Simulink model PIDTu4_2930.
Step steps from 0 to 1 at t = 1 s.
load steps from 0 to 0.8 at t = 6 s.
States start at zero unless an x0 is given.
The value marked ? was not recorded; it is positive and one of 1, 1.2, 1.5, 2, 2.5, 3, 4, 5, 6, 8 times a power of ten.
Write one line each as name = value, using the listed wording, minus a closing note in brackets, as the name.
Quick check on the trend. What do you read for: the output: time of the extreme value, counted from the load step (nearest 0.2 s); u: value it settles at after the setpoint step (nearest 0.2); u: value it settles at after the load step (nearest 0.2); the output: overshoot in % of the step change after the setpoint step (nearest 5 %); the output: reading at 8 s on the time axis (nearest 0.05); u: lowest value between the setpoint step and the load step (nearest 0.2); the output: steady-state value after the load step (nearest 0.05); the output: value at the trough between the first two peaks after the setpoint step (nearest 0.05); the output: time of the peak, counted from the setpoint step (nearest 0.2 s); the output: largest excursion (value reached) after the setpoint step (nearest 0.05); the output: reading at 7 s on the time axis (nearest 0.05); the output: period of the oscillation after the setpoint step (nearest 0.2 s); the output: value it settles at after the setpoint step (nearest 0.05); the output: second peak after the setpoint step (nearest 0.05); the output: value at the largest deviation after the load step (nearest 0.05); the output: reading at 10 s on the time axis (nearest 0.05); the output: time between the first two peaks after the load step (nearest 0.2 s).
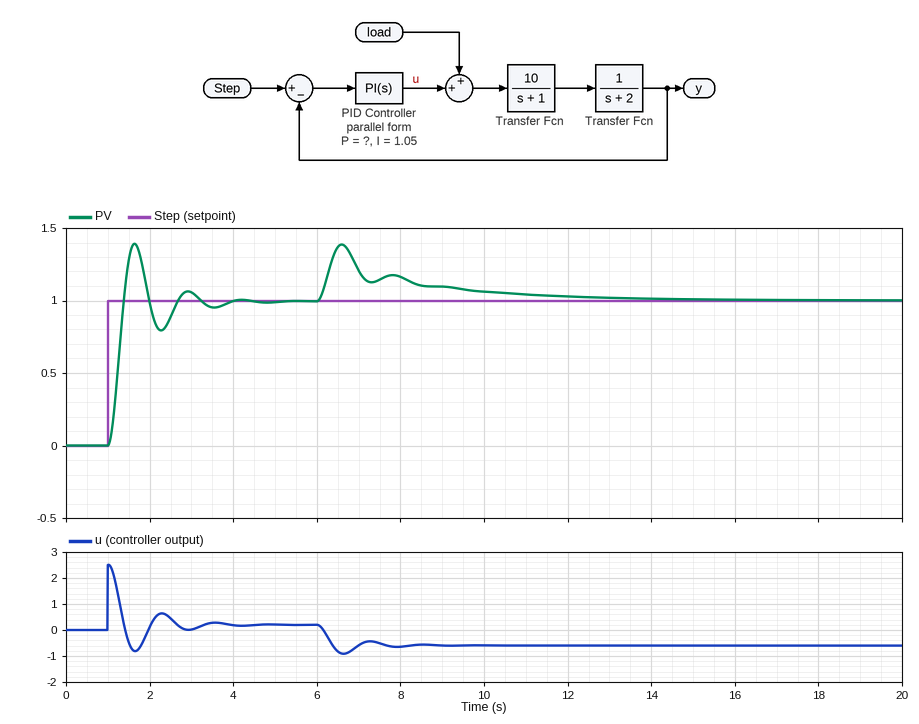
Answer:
the output: time of the extreme value, counted from the load step = 0.6 s
u: value it settles at after the setpoint step = 0.2
u: value it settles at after the load step = -0.6
the output: overshoot in % of the step change after the setpoint step = 40 %
the output: reading at 8 s on the time axis = 1.15
u: lowest value between the setpoint step and the load step = -0.8
the output: steady-state value after the load step = 1.00
the output: value at the trough between the first two peaks after the setpoint step = 0.80
the output: time of the peak, counted from the setpoint step = 0.6 s
the output: largest excursion (value reached) after the setpoint step = 1.40
the output: reading at 7 s on the time axis = 1.20
the output: period of the oscillation after the setpoint step = 1.2 s
the output: value it settles at after the setpoint step = 1.00
the output: second peak after the setpoint step = 1.05
the output: value at the largest deviation after the load step = 1.40
the output: reading at 10 s on the time axis = 1.05
the output: time between the first two peaks after the load step = 1.2 s
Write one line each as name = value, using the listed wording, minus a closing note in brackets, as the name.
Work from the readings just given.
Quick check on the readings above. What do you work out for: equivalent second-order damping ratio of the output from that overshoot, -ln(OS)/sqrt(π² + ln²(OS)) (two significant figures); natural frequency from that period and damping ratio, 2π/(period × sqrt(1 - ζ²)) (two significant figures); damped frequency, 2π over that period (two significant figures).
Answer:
equivalent second-order damping ratio of the output from that overshoot, -ln(OS)/sqrt(π² + ln²(OS)) = 0.28
natural frequency from that period and damping ratio, 2π/(period × sqrt(1 - ζ²)) = 5.5 rad/s
damped frequency, 2π over that period = 5.2 rad/s
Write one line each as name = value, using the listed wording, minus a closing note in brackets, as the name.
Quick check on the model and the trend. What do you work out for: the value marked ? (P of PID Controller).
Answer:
the value marked ? = 2.5
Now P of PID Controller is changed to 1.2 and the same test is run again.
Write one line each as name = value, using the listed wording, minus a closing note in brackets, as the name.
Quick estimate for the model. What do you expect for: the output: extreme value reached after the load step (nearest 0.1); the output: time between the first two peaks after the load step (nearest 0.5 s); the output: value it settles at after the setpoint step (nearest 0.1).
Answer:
the output: extreme value reached after the load step = 1.6
the output: time between the first two peaks after the load step = 2.0 s
the output: value it settles at after the setpoint step = 1.0
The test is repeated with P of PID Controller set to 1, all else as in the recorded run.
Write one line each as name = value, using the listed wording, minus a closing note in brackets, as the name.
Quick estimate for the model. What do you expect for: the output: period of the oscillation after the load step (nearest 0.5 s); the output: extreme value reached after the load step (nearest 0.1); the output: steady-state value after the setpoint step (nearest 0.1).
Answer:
the output: period of the oscillation after the load step = 2.0 s
the output: extreme value reached after the load step = 1.7
the output: steady-state value after the setpoint step = 1.0
